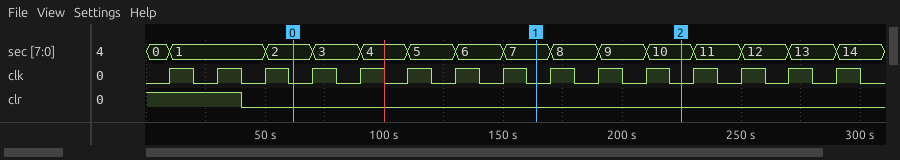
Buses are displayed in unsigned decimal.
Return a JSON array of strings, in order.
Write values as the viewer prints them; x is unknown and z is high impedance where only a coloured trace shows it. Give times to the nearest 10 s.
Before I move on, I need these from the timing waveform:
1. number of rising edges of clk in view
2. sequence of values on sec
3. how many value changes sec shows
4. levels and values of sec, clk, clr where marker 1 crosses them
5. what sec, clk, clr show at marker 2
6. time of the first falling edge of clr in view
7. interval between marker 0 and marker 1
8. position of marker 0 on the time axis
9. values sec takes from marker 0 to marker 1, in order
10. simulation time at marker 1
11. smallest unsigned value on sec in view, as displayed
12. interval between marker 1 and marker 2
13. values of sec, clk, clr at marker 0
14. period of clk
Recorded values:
["15", "0, 1, 2, 3, 4, 5, 6, 7, 8, 9, 10, 11, 12, 13, 14", "14", "sec=7, clk=0, clr=0", "sec=10, clk=0, clr=0", "40 s", "100 s", "60 s", "2, 3, 4, 5, 6, 7", "160 s", "0", "60 s", "sec=2, clk=0, clr=0", "20 s"]
